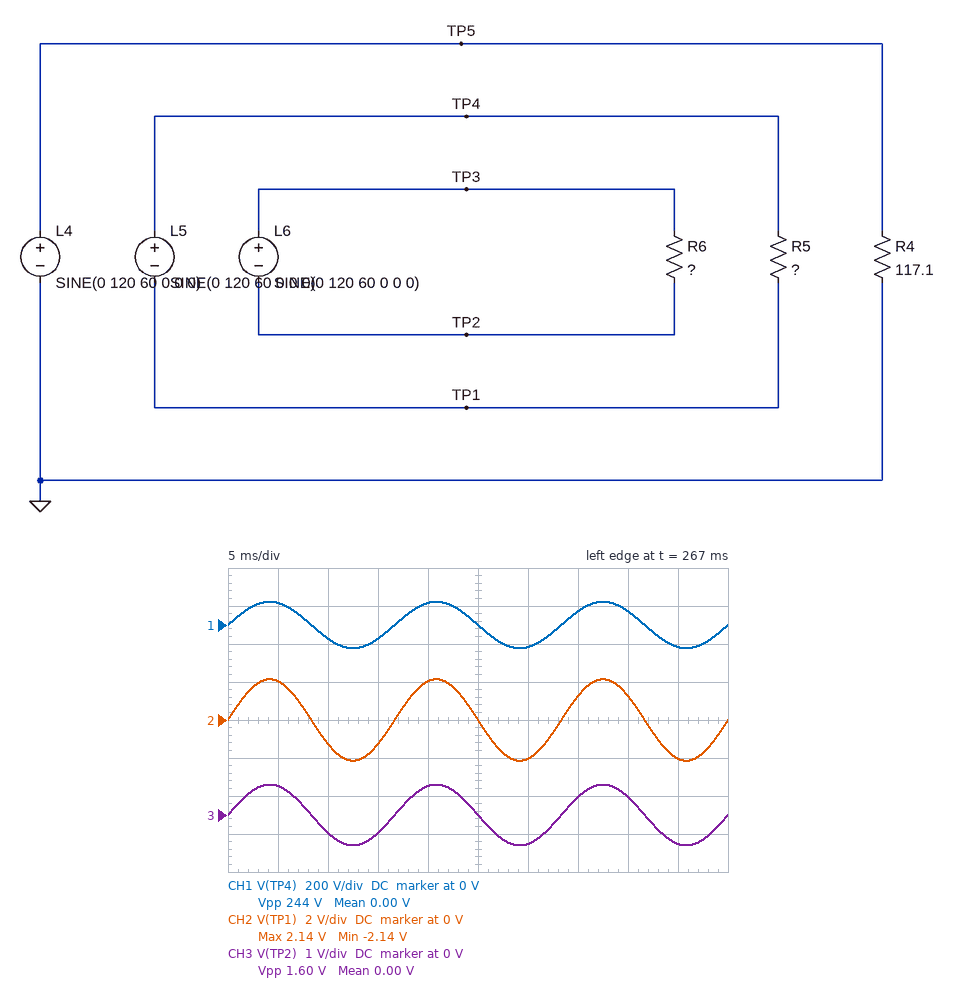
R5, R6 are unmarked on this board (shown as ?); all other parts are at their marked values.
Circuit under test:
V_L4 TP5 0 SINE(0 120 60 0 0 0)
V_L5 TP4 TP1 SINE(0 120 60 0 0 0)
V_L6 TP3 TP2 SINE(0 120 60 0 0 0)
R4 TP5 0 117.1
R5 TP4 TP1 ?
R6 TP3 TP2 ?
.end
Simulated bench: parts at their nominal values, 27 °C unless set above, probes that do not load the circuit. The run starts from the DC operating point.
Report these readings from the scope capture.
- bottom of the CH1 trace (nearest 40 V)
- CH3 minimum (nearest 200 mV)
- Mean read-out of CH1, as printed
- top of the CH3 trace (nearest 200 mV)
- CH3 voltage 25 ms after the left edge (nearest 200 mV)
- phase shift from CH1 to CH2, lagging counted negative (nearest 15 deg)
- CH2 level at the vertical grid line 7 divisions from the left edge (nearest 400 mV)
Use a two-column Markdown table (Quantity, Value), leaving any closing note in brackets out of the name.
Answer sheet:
| Quantity | Value |
|---|---|
| bottom of the CH1 trace | -120 V |
| CH3 minimum | -800 mV |
| Mean read-out of CH1, as printed | 0.00 V |
| top of the CH3 trace | 800 mV |
| CH3 voltage 25 ms after the left edge | 0 V |
| phase shift from CH1 to CH2, lagging counted negative | 0 deg |
| CH2 level at the vertical grid line 7 divisions from the left edge | 1.2 V |
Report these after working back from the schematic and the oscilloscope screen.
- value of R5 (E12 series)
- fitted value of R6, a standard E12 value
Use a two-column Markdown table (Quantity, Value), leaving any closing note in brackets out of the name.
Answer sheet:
| Quantity | Value |
|---|---|
| value of R5 | 56 Ω |
| fitted value of R6, a standard E12 value | 150 Ω |
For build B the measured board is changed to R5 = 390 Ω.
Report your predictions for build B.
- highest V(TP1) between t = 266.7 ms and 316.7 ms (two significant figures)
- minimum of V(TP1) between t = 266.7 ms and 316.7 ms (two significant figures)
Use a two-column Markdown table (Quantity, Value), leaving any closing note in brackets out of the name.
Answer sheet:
| Quantity | Value |
|---|---|
| highest V(TP1) between t = 266.7 ms and 316.7 ms | 310 mV |
| minimum of V(TP1) between t = 266.7 ms and 316.7 ms | -310 mV |
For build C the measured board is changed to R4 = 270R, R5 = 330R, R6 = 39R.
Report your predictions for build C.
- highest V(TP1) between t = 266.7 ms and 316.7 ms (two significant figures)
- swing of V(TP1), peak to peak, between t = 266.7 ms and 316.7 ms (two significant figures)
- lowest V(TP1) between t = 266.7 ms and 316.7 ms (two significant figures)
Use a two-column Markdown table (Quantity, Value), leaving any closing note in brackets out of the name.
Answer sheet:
| Quantity | Value |
|---|---|
| highest V(TP1) between t = 266.7 ms and 316.7 ms | 360 mV |
| swing of V(TP1), peak to peak, between t = 266.7 ms and 316.7 ms | 730 mV |
| lowest V(TP1) between t = 266.7 ms and 316.7 ms | -360 mV |
